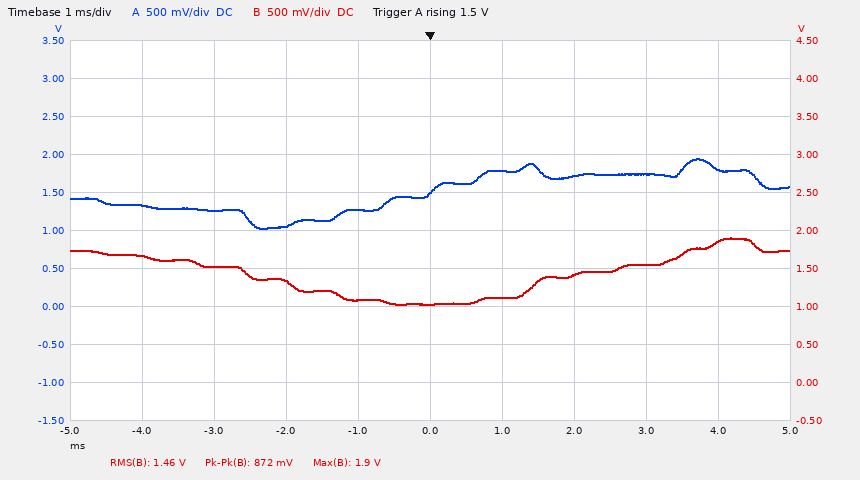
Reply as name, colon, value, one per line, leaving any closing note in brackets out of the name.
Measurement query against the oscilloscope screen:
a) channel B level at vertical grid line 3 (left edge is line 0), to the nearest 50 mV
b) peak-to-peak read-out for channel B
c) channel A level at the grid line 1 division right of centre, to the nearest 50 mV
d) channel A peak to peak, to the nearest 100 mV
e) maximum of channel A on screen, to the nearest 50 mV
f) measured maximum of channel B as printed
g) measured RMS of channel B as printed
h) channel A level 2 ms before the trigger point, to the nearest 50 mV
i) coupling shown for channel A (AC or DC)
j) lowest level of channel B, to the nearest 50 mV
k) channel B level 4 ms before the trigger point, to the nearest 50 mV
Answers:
channel B level at vertical grid line 3 (left edge is line 0), to the nearest 50 mV: 1.35 V
peak-to-peak read-out for channel B: 872 mV
channel A level at the grid line 1 division right of centre, to the nearest 50 mV: 1.80 V
channel A peak to peak, to the nearest 100 mV: 900 mV
maximum of channel A on screen, to the nearest 50 mV: 1.95 V
measured maximum of channel B as printed: 1.9 V
measured RMS of channel B as printed: 1.46 V
channel A level 2 ms before the trigger point, to the nearest 50 mV: 1.05 V
coupling shown for channel A: DC
lowest level of channel B, to the nearest 50 mV: 1.05 V
channel B level 4 ms before the trigger point, to the nearest 50 mV: 1.65 V
